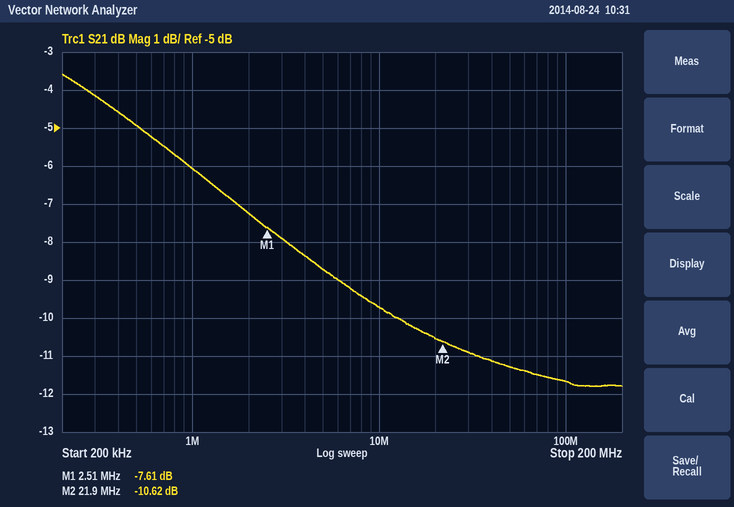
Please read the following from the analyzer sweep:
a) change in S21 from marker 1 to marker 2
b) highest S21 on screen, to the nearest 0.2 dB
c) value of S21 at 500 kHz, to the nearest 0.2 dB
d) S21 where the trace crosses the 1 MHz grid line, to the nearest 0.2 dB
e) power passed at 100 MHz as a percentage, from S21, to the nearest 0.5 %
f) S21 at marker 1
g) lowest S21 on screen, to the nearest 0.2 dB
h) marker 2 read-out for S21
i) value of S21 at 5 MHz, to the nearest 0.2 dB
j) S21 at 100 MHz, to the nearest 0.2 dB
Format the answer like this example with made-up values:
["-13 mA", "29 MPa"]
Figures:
["-3.01 dB", "-3.6 dB", "-5.0 dB", "-6.0 dB", "7.0 %", "-7.61 dB", "-11.8 dB", "-10.62 dB", "-8.8 dB", "-11.6 dB"]
